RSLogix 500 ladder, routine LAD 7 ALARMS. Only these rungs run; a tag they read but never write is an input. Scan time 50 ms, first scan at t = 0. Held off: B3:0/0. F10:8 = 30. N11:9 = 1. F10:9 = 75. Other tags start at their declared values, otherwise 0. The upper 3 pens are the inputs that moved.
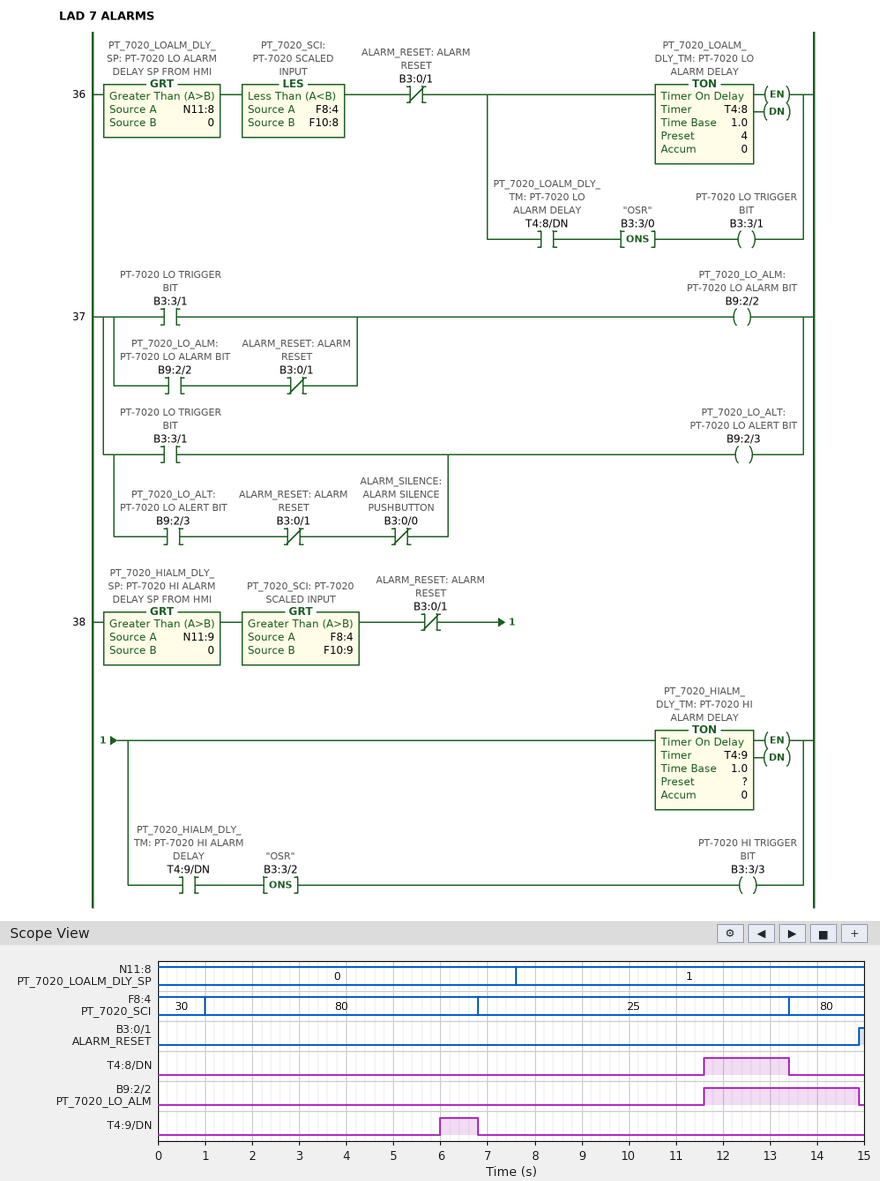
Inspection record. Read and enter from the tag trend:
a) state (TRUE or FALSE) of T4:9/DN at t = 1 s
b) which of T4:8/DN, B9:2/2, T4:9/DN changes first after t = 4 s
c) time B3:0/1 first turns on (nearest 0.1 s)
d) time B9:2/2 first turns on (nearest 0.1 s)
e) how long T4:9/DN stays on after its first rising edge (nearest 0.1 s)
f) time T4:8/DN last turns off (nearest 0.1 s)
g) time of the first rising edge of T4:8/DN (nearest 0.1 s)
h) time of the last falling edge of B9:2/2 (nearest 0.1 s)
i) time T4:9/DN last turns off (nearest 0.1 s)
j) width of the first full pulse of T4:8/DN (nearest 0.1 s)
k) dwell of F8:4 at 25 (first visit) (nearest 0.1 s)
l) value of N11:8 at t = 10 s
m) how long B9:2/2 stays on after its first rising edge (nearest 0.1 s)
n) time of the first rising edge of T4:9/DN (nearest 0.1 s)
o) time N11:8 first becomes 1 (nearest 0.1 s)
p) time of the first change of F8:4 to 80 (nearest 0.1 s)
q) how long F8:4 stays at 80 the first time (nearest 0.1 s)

FALSE
T4:9/DN
14.9 s
11.6 s
0.8 s
13.4 s
11.6 s
14.9 s
6.8 s
1.8 s
6.6 s
1
3.3 s
6.0 s
7.6 s
1.0 s
5.8 s
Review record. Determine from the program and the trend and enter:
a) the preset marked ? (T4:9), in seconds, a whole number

5 s
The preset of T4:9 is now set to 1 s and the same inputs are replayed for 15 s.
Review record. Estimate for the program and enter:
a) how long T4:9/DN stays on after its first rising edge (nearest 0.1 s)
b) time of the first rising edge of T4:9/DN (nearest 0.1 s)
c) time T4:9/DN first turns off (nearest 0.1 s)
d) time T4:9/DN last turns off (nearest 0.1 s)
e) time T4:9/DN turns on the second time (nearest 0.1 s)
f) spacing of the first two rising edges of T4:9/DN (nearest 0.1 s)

4.8 s
2.0 s
6.8 s
14.9 s
14.4 s
12.4 s
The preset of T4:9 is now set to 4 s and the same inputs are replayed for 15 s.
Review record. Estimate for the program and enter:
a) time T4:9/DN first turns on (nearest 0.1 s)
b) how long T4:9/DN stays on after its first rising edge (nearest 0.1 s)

5.0 s
1.8 s
